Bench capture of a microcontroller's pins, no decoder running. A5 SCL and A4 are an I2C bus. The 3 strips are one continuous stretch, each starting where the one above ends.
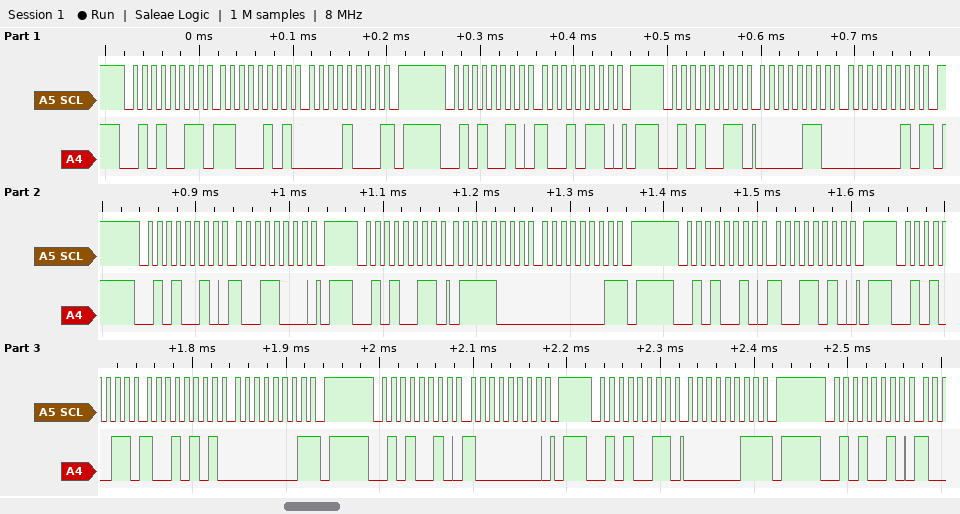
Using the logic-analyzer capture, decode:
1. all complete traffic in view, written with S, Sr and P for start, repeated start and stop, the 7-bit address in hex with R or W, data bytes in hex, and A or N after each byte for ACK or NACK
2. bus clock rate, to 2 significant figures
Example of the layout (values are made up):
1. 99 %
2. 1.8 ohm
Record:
1. S 29R A C5 A 08 N P S 29W A 96 A P S 29R A 06 A 02 N P S 29W A 98 A P S 29R A 78 A 01 N P S 29W A 9A A P S 29R A 95 A 01 N P S 29W A 80 A P S 29R A 03 N P S 29W A
2. 100 kHz
